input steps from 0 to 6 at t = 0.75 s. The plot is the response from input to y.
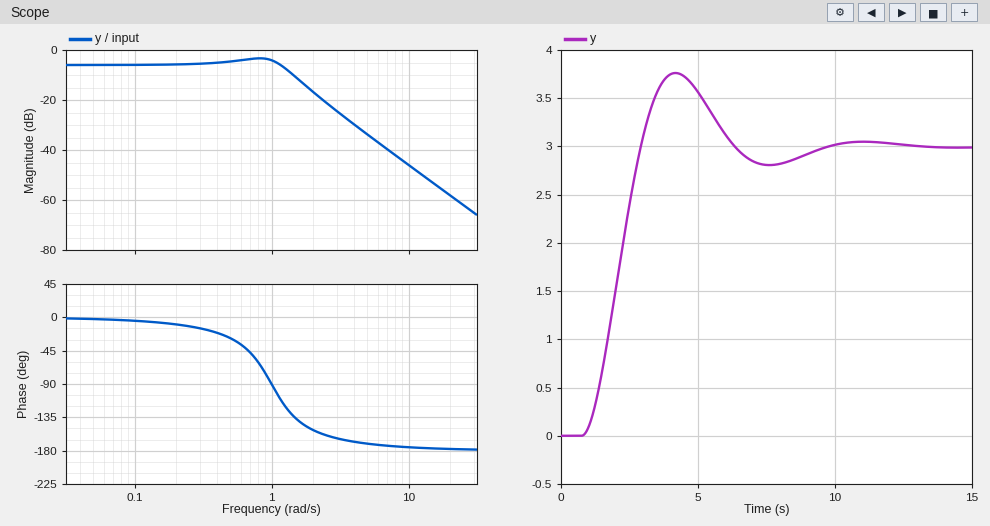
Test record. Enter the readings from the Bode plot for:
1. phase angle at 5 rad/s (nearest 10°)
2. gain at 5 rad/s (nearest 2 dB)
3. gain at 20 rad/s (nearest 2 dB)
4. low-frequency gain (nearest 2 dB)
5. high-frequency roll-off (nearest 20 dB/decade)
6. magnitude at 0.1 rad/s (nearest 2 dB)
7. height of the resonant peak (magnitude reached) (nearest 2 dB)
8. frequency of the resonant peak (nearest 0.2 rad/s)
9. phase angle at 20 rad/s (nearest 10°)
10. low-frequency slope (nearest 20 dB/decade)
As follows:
-170°
-34 dB
-58 dB
-6 dB
-40 dB/decade
-6 dB
-4 dB
0.8 rad/s
-180°
0 dB/decade
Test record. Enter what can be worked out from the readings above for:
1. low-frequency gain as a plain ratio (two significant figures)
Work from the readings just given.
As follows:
0.50
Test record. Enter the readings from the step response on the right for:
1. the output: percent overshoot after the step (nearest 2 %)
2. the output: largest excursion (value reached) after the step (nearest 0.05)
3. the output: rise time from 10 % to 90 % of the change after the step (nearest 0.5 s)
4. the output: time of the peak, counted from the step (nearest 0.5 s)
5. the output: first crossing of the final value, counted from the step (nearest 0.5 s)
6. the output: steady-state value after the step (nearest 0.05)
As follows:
26 %
3.75
1.5 s
3.5 s
2.0 s
3.00
